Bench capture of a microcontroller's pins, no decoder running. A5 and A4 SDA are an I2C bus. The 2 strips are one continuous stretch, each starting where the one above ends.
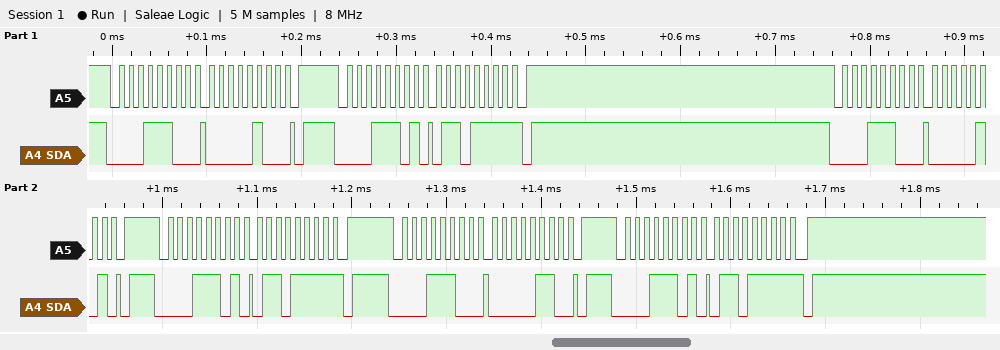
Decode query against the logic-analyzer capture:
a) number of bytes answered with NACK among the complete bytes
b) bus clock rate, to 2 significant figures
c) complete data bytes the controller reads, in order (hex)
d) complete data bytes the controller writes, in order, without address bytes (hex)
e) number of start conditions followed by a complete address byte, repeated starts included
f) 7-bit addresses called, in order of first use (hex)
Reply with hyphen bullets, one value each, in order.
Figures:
- 3
- 100 kHz
- 6F 6F 6F
- 04 05 06
- 6
- 0x0E
